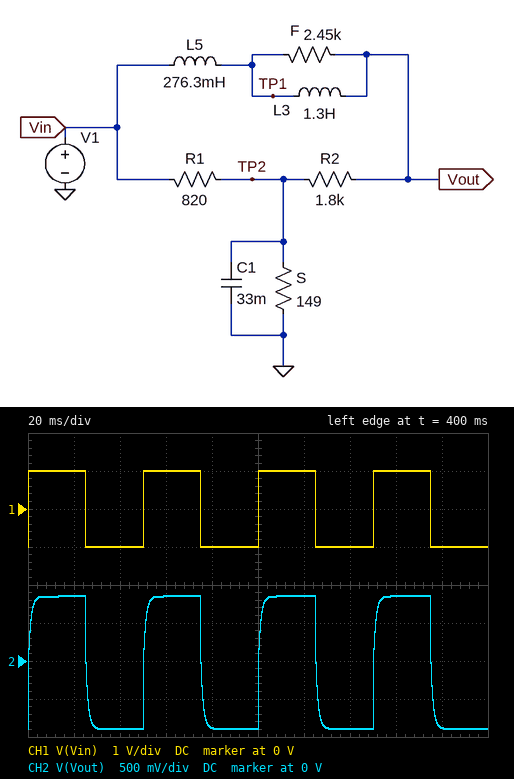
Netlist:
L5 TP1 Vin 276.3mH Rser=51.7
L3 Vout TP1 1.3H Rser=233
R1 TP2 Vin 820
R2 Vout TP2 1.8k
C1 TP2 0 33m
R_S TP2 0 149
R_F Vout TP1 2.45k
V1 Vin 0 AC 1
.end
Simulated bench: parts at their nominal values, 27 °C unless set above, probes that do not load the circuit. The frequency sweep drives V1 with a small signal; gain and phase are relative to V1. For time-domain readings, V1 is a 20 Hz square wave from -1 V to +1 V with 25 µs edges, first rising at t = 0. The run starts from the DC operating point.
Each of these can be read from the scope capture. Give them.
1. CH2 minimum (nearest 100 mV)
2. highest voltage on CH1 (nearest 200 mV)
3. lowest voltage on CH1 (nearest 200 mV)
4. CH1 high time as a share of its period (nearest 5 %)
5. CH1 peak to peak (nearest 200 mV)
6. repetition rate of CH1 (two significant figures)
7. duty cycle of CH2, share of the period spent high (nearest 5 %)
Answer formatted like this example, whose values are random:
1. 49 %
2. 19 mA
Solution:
1. -900 mV
2. 1.0 V
3. -1.0 V
4. 50 %
5. 2.0 V
6. 20 Hz
7. 50 %
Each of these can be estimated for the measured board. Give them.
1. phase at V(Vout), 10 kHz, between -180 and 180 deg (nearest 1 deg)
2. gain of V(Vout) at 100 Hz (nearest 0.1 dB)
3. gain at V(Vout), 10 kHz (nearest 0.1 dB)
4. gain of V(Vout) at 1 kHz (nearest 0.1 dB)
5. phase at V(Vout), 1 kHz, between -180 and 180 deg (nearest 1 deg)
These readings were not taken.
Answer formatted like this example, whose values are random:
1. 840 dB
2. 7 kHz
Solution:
1. -76 deg
2. -2.5 dB
3. -20.0 dB
4. -8.4 dB
5. -30 deg
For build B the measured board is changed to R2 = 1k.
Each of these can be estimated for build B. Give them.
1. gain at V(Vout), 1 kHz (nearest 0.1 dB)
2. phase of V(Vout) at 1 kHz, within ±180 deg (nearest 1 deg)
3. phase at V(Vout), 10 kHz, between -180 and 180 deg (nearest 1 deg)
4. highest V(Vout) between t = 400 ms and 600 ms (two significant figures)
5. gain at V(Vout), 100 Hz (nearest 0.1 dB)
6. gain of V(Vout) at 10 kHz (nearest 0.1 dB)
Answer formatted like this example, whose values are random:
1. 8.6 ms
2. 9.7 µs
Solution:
1. -12.2 dB
2. -36 deg
3. -79 deg
4. 750 mV
5. -4.4 dB
6. -25.0 dB
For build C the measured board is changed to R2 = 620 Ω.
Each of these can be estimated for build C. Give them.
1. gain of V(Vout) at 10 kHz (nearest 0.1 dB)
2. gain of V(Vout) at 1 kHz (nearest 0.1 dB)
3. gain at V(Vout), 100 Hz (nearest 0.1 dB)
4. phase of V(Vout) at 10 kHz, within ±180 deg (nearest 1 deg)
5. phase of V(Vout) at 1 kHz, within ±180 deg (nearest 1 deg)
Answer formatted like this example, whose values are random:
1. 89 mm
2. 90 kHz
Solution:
1. -29.1 dB
2. -15.7 dB
3. -6.7 dB
4. -80 deg
5. -40 deg
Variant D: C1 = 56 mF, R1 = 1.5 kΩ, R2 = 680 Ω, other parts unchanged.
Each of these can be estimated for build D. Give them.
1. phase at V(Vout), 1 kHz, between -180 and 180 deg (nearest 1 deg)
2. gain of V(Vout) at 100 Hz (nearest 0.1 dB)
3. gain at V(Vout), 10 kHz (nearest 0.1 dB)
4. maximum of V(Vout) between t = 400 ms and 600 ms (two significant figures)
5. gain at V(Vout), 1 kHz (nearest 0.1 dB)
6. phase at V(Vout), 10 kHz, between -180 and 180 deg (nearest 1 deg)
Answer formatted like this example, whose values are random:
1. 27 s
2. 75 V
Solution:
1. -39 deg
2. -6.2 dB
3. -28.3 dB
4. 670 mV
5. -15.0 dB
6. -80 deg
